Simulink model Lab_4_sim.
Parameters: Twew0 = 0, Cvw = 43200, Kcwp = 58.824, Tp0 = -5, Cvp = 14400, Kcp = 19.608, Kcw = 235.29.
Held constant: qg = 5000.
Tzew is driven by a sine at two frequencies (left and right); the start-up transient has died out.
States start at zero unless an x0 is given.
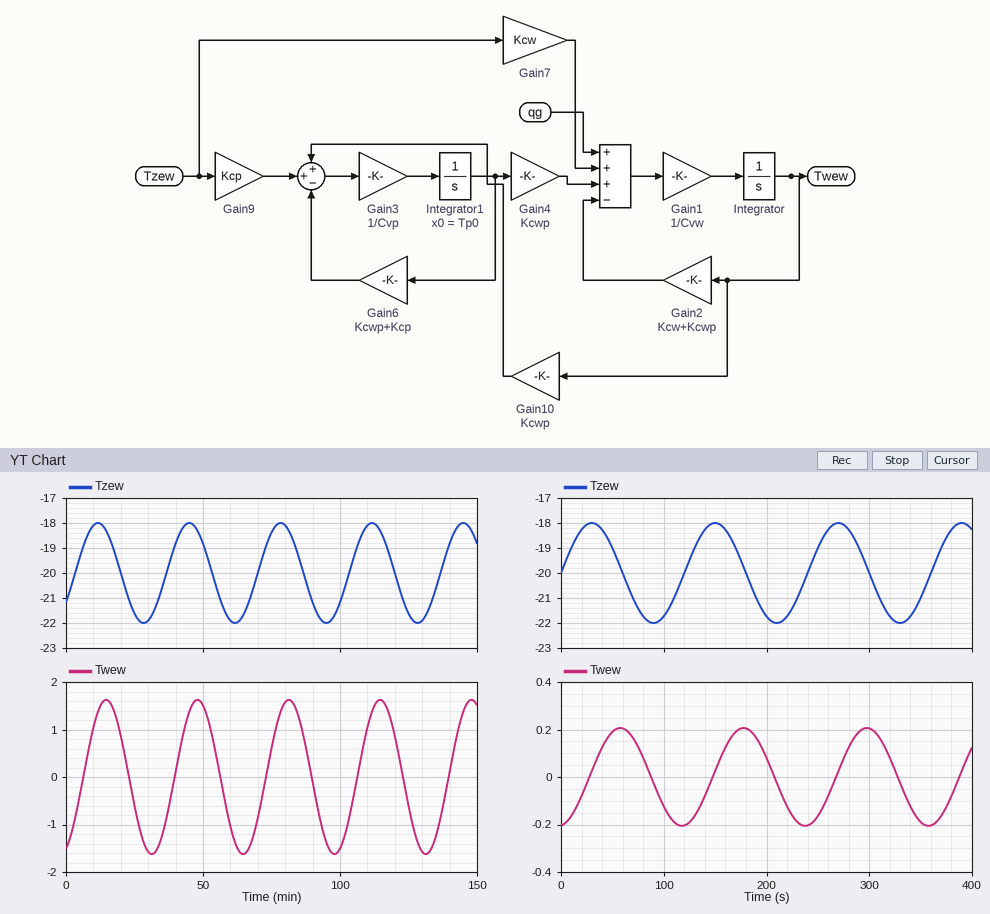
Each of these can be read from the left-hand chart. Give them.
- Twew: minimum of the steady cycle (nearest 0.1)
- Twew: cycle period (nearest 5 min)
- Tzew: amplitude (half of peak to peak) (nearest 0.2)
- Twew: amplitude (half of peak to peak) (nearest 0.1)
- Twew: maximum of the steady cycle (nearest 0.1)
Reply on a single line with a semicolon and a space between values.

-1.6; 35 min; 2.0; 1.6; 1.6
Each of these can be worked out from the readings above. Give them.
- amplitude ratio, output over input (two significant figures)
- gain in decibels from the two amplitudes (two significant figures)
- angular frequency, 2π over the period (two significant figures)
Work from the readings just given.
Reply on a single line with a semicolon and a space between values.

0.80; -1.9 dB; 0.18 rad/min
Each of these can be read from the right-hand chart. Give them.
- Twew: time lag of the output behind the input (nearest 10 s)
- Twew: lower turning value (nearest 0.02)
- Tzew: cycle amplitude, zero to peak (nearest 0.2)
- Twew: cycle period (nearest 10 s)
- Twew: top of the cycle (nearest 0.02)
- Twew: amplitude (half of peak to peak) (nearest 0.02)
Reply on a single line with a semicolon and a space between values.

30 s; -0.20; 2.0; 120 s; 0.20; 0.20
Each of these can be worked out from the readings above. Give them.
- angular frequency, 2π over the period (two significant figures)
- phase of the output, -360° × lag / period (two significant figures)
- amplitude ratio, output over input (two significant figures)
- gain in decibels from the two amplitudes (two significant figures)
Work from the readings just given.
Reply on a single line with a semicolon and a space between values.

0.052 rad/s; -90°; 0.10; -20 dB
